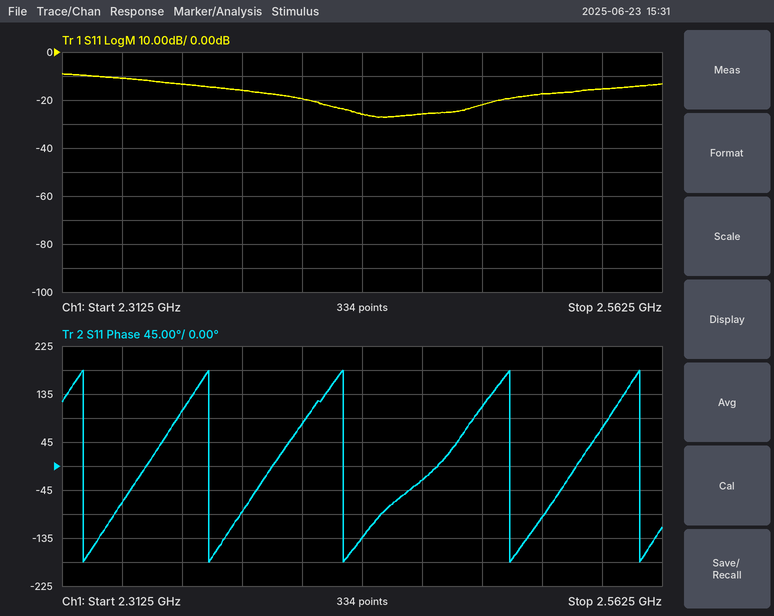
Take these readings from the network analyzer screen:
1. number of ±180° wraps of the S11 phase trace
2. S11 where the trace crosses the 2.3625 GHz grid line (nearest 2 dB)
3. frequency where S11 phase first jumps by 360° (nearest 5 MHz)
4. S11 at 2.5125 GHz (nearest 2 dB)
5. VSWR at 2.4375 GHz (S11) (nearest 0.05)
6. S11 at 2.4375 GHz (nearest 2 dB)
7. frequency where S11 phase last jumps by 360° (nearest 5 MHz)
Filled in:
5
-14 dB
2.320 GHz
-18 dB
1.10
-26 dB
2.555 GHz
